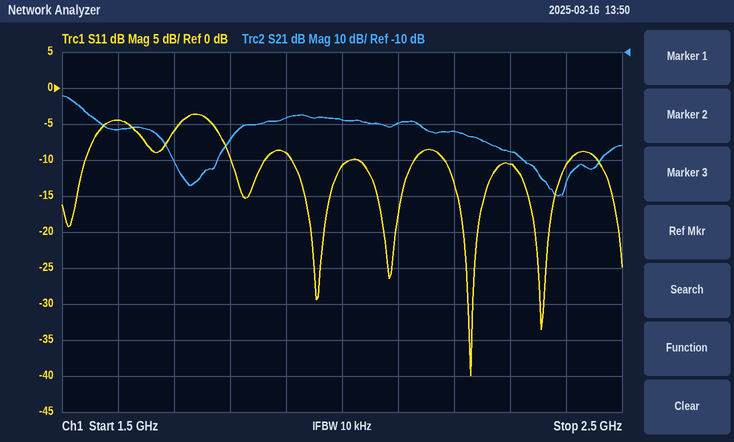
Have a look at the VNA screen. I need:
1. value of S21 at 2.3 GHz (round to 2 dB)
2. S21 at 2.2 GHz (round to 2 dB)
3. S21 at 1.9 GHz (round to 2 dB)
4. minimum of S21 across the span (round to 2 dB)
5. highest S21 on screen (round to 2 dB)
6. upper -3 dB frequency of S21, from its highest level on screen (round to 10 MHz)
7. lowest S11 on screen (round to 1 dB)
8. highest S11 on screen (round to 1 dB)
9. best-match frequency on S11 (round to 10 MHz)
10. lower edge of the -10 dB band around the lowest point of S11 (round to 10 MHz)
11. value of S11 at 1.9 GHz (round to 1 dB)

-38 dB
-32 dB
-28 dB
-50 dB
-22 dB
1.53 GHz
-40 dB
-4 dB
2.23 GHz
2.18 GHz
-9 dB
